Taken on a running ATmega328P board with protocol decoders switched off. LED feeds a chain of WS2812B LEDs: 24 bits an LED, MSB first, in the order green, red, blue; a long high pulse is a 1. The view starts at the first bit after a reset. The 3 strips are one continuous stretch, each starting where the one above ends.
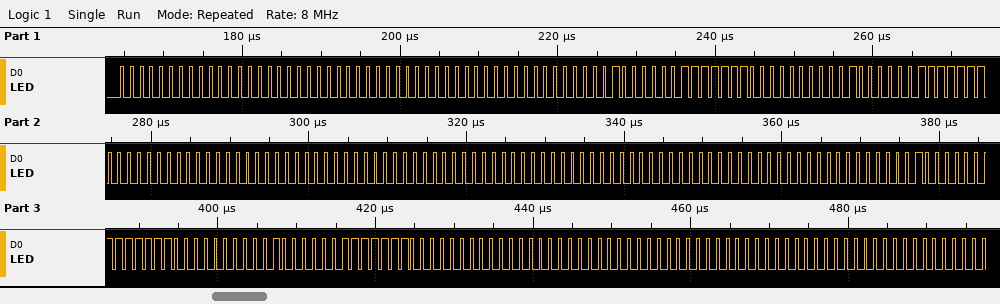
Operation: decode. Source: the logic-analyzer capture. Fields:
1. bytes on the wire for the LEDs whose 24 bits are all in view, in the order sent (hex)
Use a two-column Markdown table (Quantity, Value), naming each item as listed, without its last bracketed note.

| Quantity | Value |
|---|---|
| bytes on the wire for the LEDs whose 24 bits are all in view, in the order sent | 00 00 00 00 00 00 20 7F 00 20 7F 00 00 00 00 00 00 00 00 00 00 20 7F 00 20 7F 00 00 00 00 00 00 00 |
